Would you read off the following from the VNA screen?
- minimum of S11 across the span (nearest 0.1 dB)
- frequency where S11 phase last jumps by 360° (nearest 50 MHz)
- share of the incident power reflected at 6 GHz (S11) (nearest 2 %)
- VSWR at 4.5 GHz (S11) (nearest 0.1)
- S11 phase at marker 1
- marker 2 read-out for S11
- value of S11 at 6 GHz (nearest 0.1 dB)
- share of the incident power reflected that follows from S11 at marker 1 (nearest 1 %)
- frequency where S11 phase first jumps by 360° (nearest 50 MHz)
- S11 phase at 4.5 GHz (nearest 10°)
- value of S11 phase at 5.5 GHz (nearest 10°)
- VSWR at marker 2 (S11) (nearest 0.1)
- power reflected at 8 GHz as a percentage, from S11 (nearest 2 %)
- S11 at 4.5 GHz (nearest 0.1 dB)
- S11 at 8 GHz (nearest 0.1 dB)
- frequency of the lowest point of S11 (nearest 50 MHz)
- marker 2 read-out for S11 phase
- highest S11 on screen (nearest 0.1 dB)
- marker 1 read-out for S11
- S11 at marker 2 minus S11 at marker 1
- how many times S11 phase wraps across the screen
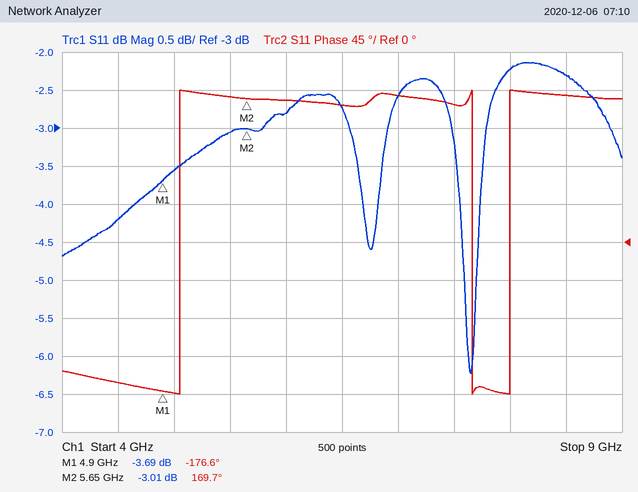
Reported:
-6.2 dB
8.00 GHz
52 %
4.2
-176.6°
-3.01 dB
-2.8 dB
43 %
5.05 GHz
-170°
170°
5.8
60 %
-4.2 dB
-2.2 dB
7.65 GHz
169.7°
-2.1 dB
-3.69 dB
0.68 dB
3
